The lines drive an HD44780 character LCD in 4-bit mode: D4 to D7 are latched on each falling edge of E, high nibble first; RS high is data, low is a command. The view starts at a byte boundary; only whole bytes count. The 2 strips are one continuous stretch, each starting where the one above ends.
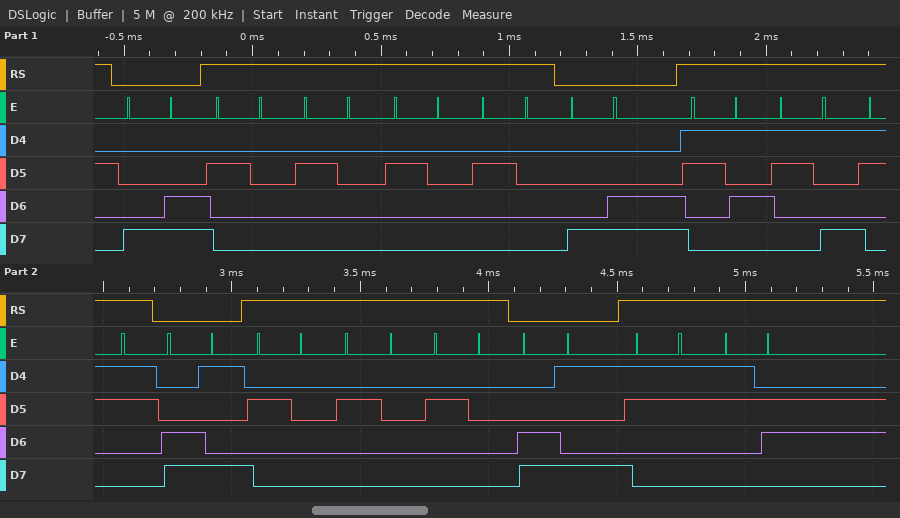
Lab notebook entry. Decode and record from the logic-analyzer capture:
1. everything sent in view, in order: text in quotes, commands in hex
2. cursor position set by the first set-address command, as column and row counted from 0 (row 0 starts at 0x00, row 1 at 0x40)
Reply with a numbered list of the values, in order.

1. 0x8C "    " 0x8C "593" 0xC9 "   " 0xC9 "36"
2. column 12, row 0
